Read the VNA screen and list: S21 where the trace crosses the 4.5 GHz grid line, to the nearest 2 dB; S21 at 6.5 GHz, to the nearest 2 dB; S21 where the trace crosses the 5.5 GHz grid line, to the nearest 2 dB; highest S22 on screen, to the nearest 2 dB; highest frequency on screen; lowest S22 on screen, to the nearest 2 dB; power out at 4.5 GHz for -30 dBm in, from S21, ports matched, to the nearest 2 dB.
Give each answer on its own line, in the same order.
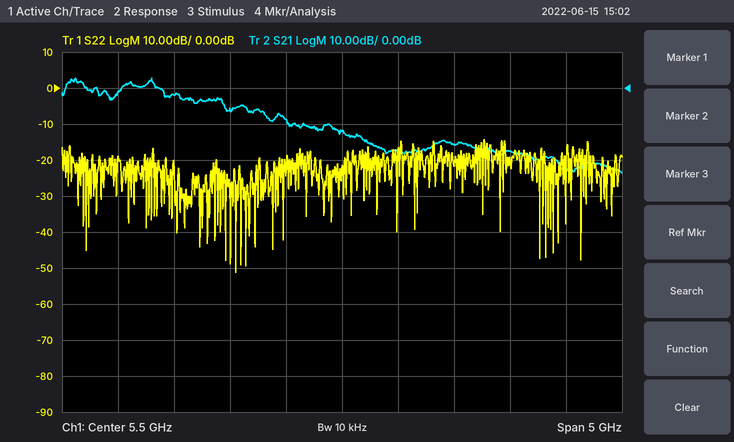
-6 dB
-16 dB
-12 dB
-14 dB
8 GHz
-52 dB
-36 dBm
